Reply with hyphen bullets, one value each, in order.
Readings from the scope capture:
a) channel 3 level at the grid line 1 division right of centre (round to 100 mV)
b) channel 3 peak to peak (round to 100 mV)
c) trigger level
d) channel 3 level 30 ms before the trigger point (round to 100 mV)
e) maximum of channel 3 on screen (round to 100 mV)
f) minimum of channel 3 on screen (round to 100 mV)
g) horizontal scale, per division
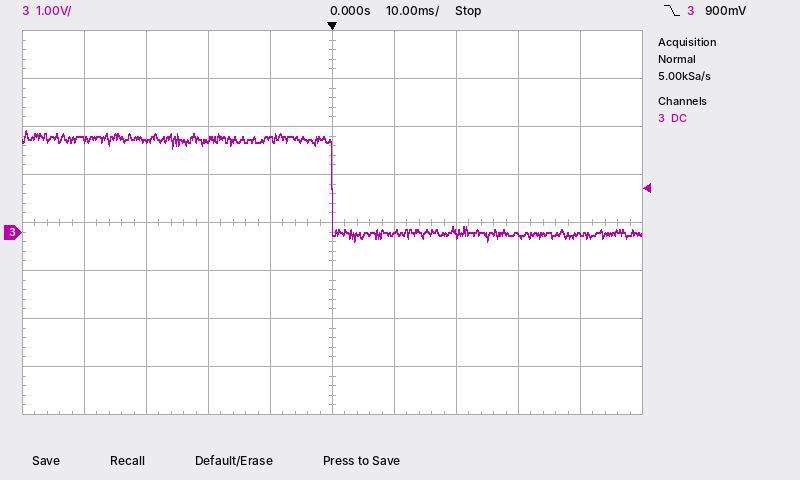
- 0.0 V
- 2.3 V
- 900 mV
- 1.9 V
- 2.1 V
- -200 mV
- 10 ms
